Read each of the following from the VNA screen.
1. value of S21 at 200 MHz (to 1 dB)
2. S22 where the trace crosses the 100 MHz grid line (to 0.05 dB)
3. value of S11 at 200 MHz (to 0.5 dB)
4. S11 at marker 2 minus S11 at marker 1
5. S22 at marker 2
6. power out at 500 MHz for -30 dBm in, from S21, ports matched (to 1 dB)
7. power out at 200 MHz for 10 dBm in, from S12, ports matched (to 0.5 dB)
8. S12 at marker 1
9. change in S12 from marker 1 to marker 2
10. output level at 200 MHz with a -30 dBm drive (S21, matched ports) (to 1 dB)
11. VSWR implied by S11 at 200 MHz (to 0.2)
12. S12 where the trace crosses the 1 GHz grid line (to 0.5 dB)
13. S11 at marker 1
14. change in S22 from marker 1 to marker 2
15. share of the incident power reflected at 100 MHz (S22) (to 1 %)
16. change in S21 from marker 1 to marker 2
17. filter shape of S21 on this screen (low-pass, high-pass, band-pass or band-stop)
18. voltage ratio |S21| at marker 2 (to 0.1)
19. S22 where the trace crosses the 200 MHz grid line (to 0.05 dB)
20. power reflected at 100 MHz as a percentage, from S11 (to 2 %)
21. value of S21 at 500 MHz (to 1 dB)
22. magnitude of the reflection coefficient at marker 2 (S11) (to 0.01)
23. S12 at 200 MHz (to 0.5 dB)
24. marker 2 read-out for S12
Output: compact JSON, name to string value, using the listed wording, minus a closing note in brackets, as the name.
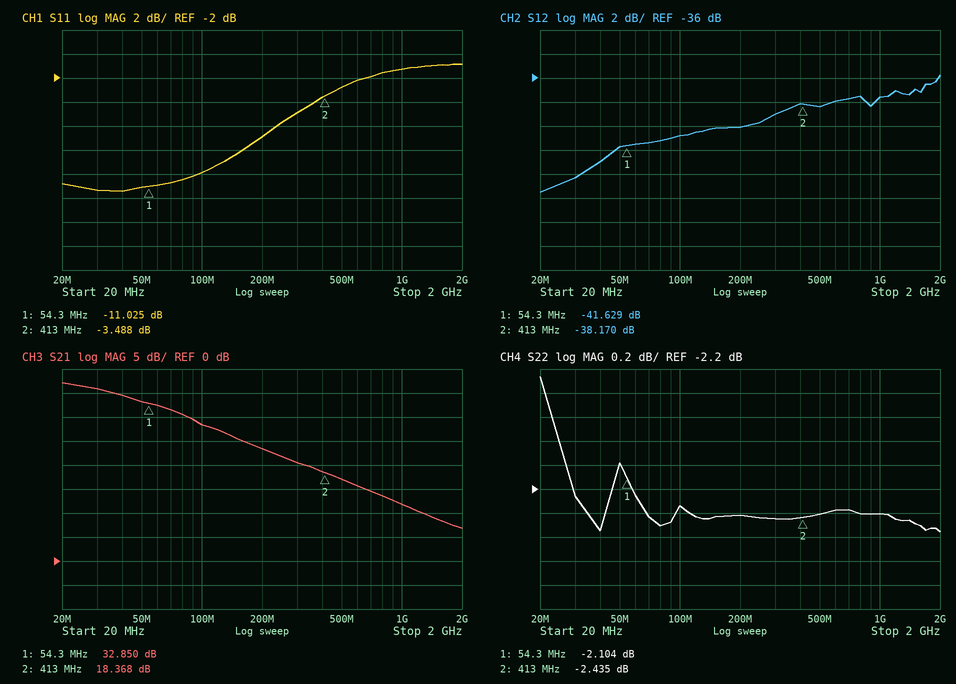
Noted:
{"value of S21 at 200 MHz": "23 dB", "S22 where the trace crosses the 100 MHz grid line": "-2.35 dB", "value of S11 at 200 MHz": "-7.0 dB", "S11 at marker 2 minus S11 at marker 1": "7.537 dB", "S22 at marker 2": "-2.435 dB", "power out at 500 MHz for -30 dBm in, from S21, ports matched": "-13 dBm", "power out at 200 MHz for 10 dBm in, from S12, ports matched": "-30.0 dBm", "S12 at marker 1": "-41.629 dB", "change in S12 from marker 1 to marker 2": "3.459 dB", "output level at 200 MHz with a -30 dBm drive (S21, matched ports)": "-7 dBm", "VSWR implied by S11 at 200 MHz": "2.6", "S12 where the trace crosses the 1 GHz grid line": "-37.5 dB", "S11 at marker 1": "-11.025 dB", "change in S22 from marker 1 to marker 2": "-0.331 dB", "share of the incident power reflected at 100 MHz (S22)": "58 %", "change in S21 from marker 1 to marker 2": "-14.482 dB", "filter shape of S21 on this screen": "low-pass", "voltage ratio |S21| at marker 2": "8.3", "S22 where the trace crosses the 200 MHz grid line": "-2.40 dB", "power reflected at 100 MHz as a percentage, from S11": "10 %", "value of S21 at 500 MHz": "17 dB", "magnitude of the reflection coefficient at marker 2 (S11)": "0.67", "S12 at 200 MHz": "-40.0 dB", "marker 2 read-out for S12": "-38.170 dB"}
